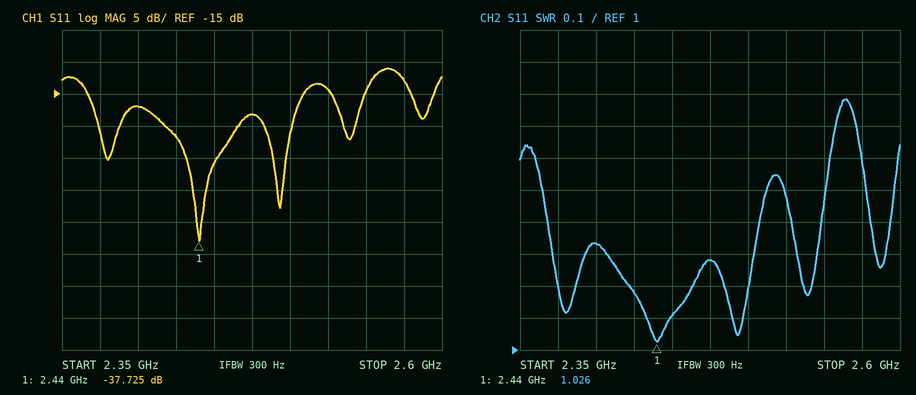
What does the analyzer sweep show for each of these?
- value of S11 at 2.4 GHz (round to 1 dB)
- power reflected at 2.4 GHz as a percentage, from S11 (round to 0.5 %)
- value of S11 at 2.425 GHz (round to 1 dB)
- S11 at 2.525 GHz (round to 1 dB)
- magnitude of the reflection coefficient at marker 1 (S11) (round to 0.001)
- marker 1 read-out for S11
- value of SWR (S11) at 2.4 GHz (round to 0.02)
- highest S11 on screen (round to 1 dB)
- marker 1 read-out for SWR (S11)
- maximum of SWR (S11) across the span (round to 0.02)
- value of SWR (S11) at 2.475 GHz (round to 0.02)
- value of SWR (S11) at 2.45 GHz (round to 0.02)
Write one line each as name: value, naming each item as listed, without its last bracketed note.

value of S11 at 2.4 GHz: -17 dB
power reflected at 2.4 GHz as a percentage, from S11: 2.0 %
value of S11 at 2.425 GHz: -22 dB
S11 at 2.525 GHz: -14 dB
magnitude of the reflection coefficient at marker 1 (S11): 0.013
marker 1 read-out for S11: -37.725 dB
value of SWR (S11) at 2.4 GHz: 1.34
highest S11 on screen: -11 dB
marker 1 read-out for SWR: 1.026
maximum of SWR (S11) across the span: 1.78
value of SWR (S11) at 2.475 GHz: 1.28
value of SWR (S11) at 2.45 GHz: 1.10
